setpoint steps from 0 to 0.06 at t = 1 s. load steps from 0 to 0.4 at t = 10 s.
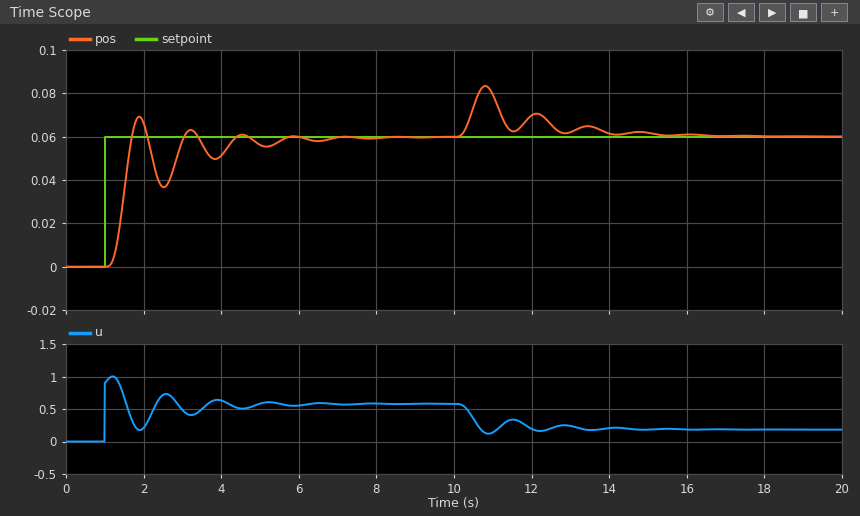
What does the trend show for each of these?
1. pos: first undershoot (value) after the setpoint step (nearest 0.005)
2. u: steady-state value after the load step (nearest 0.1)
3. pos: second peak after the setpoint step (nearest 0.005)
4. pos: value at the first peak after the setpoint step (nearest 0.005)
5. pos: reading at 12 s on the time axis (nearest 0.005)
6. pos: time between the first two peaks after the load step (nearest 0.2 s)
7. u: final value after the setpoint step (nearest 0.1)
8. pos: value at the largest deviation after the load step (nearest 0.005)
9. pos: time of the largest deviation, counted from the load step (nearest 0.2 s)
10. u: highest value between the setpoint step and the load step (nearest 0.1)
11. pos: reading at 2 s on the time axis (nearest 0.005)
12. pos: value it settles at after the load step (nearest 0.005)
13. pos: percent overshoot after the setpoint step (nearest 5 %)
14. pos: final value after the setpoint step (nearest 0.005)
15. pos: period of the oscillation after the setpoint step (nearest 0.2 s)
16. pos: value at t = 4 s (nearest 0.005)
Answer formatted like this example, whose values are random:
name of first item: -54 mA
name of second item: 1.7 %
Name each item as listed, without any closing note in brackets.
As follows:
pos: first undershoot (value) after the setpoint step: 0.035
u: steady-state value after the load step: 0.2
pos: second peak after the setpoint step: 0.065
pos: value at the first peak after the setpoint step: 0.070
pos: reading at 12 s on the time axis: 0.070
pos: time between the first two peaks after the load step: 1.4 s
u: final value after the setpoint step: 0.6
pos: value at the largest deviation after the load step: 0.085
pos: time of the largest deviation, counted from the load step: 0.8 s
u: highest value between the setpoint step and the load step: 1.0
pos: reading at 2 s on the time axis: 0.065
pos: value it settles at after the load step: 0.060
pos: percent overshoot after the setpoint step: 15 %
pos: final value after the setpoint step: 0.060
pos: period of the oscillation after the setpoint step: 1.4 s
pos: value at t = 4 s: 0.050
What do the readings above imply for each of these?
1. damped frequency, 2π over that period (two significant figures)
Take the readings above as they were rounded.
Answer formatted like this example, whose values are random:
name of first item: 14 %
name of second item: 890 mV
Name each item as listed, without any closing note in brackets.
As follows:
damped frequency, 2π over that period: 4.5 rad/s
